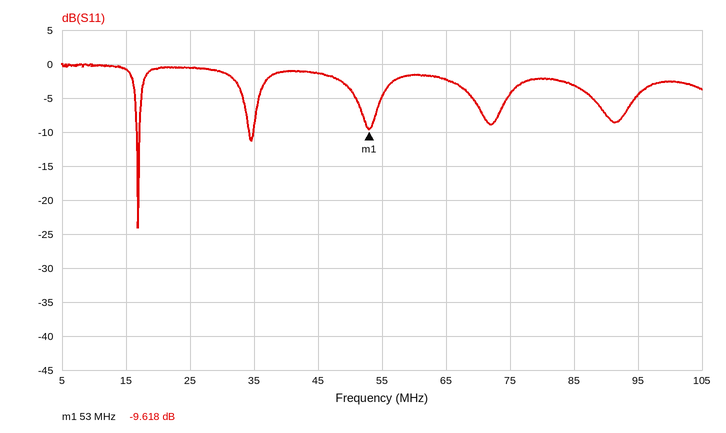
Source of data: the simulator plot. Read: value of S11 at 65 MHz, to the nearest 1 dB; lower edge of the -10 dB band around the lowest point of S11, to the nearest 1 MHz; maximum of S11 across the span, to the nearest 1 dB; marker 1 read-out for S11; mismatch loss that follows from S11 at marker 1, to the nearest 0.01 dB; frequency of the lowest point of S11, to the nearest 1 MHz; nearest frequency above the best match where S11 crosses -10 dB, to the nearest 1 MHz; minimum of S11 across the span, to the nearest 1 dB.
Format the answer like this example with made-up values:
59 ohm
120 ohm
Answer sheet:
-2 dB
17 MHz
0 dB
-9.618 dB
0.50 dB
17 MHz
17 MHz
-24 dB
